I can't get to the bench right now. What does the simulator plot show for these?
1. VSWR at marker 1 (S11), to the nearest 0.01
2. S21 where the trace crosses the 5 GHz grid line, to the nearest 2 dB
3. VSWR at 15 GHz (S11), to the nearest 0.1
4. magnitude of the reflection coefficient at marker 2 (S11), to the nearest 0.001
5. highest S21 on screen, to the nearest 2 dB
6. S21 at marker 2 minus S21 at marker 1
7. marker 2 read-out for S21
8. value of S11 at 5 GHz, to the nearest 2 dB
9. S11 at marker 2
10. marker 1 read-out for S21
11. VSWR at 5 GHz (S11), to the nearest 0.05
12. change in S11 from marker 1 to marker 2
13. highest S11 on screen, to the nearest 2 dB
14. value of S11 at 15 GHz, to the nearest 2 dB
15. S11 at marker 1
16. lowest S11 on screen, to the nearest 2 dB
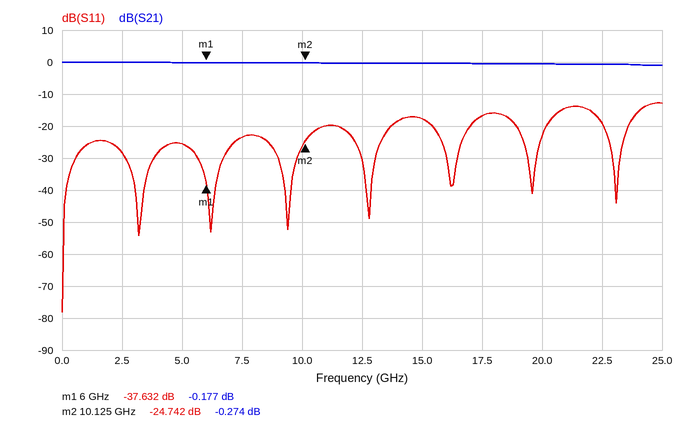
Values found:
1.03
0 dB
1.3
0.058
0 dB
-0.097 dB
-0.274 dB
-26 dB
-24.742 dB
-0.177 dB
1.10
12.890 dB
-12 dB
-18 dB
-37.632 dB
-78 dB
